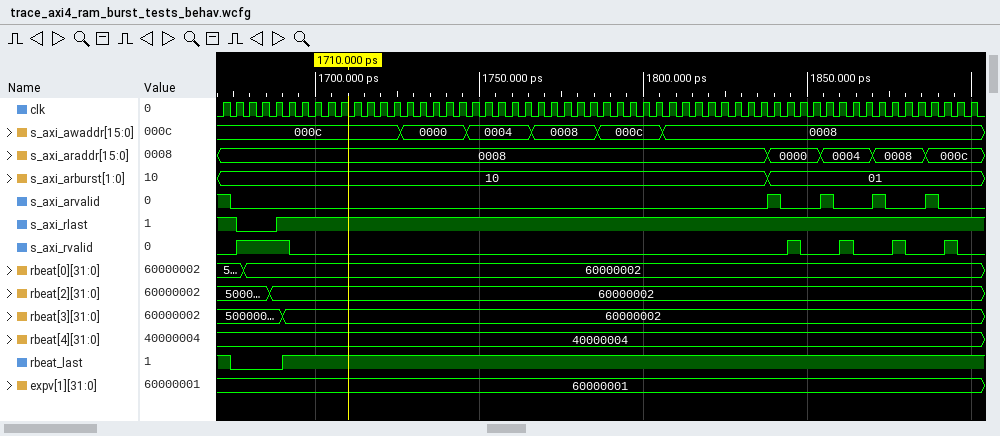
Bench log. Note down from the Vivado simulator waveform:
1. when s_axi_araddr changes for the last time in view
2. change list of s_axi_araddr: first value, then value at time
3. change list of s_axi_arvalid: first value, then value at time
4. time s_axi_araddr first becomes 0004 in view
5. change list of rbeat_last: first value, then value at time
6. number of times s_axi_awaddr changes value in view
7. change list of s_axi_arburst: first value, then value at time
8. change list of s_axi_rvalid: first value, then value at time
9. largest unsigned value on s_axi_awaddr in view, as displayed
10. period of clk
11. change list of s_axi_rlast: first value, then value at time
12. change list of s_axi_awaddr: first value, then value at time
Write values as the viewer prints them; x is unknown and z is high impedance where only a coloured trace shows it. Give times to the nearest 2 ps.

1886 ps
0008, 0000 at 1838 ps, 0004 at 1854 ps, 0008 at 1870 ps, 000c at 1886 ps
1, 0 at 1674 ps, 1 at 1838 ps, 0 at 1842 ps, 1 at 1854 ps, 0 at 1858 ps, 1 at 1870 ps, 0 at 1874 ps, 1 at 1886 ps, 0 at 1890 ps
1854 ps
1, 0 at 1674 ps, 1 at 1690 ps
5
10, 01 at 1838 ps
0, 1 at 1676 ps, 0 at 1692 ps, 1 at 1844 ps, 0 at 1848 ps, 1 at 1860 ps, 0 at 1864 ps, 1 at 1876 ps, 0 at 1880 ps, 1 at 1892 ps, 0 at 1896 ps
000c
4 ps
1, 0 at 1676 ps, 1 at 1688 ps
000c, 0000 at 1726 ps, 0004 at 1746 ps, 0008 at 1766 ps, 000c at 1786 ps, 0008 at 1806 ps
